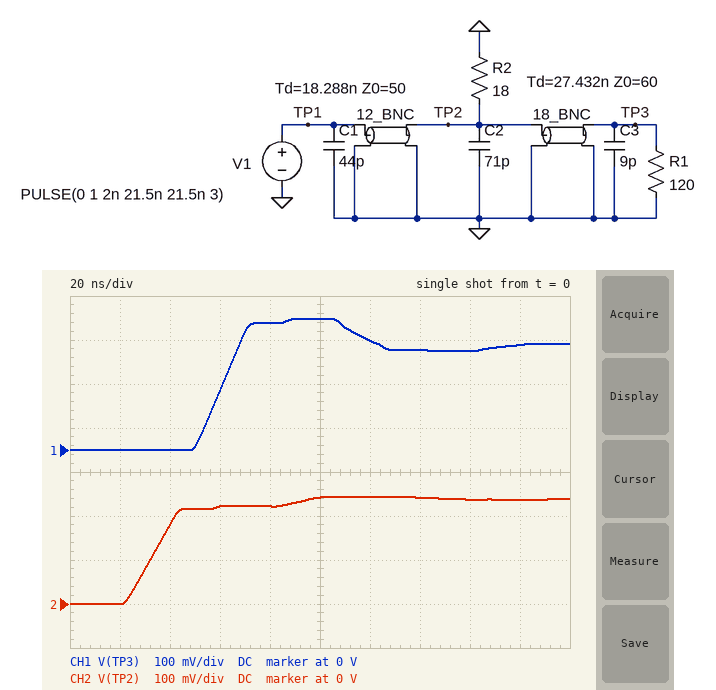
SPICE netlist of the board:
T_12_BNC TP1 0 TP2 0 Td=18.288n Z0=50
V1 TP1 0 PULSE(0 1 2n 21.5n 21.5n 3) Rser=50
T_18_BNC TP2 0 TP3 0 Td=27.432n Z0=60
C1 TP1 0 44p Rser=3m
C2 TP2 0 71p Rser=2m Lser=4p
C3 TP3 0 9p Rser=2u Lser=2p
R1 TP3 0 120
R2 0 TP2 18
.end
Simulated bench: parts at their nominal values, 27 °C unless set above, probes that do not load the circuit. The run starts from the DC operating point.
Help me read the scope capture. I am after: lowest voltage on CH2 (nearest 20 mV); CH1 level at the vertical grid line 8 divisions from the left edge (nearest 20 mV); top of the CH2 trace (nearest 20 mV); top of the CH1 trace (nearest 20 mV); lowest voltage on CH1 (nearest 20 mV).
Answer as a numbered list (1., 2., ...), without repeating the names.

1. 0 V
2. 220 mV
3. 240 mV
4. 300 mV
5. 0 V
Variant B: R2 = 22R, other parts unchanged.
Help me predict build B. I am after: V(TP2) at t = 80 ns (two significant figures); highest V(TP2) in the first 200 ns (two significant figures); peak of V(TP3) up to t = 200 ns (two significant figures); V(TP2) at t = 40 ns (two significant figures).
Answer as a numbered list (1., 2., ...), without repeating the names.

1. 250 mV
2. 280 mV
3. 330 mV
4. 200 mV
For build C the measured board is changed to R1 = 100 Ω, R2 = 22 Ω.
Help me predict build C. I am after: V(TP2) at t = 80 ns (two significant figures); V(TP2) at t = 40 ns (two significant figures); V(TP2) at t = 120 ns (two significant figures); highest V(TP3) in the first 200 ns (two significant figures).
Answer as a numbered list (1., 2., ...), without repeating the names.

1. 250 mV
2. 200 mV
3. 270 mV
4. 310 mV
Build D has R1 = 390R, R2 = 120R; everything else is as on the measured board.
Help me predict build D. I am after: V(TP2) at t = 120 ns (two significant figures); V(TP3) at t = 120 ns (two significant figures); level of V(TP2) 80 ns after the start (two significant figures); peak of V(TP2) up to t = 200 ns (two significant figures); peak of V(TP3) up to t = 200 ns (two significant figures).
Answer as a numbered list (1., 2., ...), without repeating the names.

1. 680 mV
2. 650 mV
3. 450 mV
4. 690 mV
5. 780 mV
